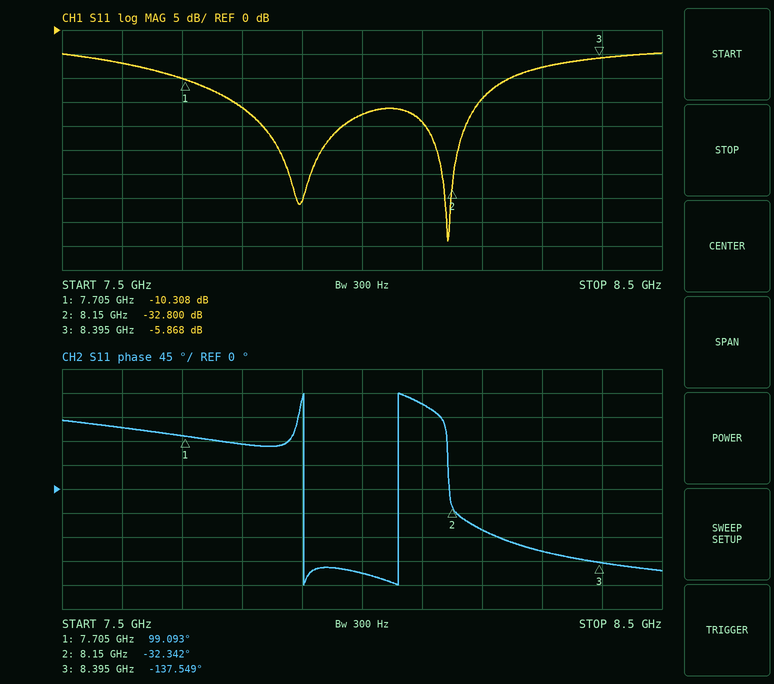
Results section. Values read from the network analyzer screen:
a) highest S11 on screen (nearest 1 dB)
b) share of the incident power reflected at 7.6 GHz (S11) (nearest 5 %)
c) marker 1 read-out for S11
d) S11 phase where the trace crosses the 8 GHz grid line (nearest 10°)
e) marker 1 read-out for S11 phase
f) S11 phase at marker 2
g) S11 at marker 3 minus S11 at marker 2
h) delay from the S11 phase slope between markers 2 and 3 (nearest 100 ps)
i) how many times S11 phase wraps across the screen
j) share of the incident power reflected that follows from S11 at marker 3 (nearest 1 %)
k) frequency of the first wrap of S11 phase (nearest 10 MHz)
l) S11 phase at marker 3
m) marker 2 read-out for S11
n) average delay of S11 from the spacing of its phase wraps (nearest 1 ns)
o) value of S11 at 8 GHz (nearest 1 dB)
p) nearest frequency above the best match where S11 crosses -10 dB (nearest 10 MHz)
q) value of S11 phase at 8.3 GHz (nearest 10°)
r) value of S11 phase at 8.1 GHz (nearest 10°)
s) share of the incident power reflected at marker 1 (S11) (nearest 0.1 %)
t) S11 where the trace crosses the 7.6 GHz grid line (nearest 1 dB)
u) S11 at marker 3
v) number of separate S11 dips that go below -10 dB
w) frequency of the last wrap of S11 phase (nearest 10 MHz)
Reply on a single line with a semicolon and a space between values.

-5 dB; 20 %; -10.308 dB; -160°; 99.093°; -32.342°; 26.932 dB; 1.2 ns; 2; 26 %; 7.90 GHz; -137.549°; -32.800 dB; 6 ns; -18 dB; 8.25 GHz; -120°; 160°; 9.3 %; -7 dB; -5.868 dB; 2; 8.06 GHz
